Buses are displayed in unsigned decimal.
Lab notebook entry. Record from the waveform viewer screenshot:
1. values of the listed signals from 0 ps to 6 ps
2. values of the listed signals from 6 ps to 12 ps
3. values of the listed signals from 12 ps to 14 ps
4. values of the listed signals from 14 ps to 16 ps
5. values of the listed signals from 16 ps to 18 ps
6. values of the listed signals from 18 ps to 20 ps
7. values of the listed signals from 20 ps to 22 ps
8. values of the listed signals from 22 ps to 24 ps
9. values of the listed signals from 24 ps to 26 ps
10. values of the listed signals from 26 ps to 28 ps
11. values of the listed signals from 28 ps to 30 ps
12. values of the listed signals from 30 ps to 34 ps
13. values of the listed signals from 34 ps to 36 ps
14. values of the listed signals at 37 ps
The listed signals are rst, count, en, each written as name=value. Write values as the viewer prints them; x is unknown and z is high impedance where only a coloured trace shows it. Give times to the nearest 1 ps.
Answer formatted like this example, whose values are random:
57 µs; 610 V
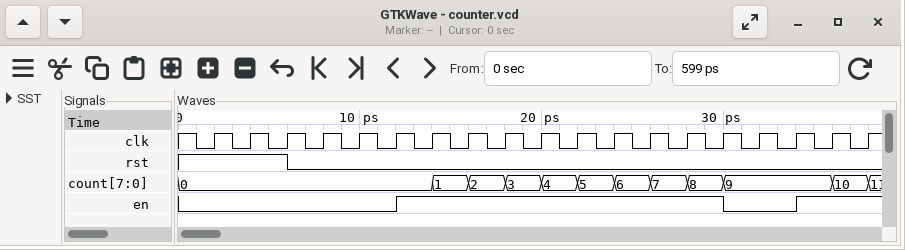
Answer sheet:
rst=1, count=0, en=0; rst=0, count=0, en=0; rst=0, count=0, en=1; rst=0, count=1, en=1; rst=0, count=2, en=1; rst=0, count=3, en=1; rst=0, count=4, en=1; rst=0, count=5, en=1; rst=0, count=6, en=1; rst=0, count=7, en=1; rst=0, count=8, en=1; rst=0, count=9, en=0; rst=0, count=9, en=1; rst=0, count=10, en=1
